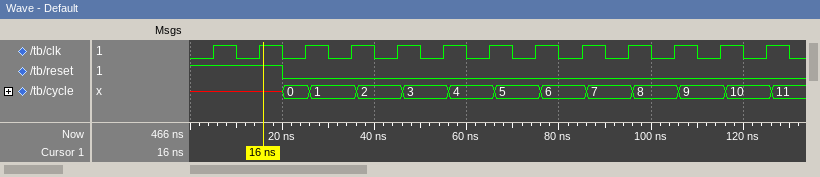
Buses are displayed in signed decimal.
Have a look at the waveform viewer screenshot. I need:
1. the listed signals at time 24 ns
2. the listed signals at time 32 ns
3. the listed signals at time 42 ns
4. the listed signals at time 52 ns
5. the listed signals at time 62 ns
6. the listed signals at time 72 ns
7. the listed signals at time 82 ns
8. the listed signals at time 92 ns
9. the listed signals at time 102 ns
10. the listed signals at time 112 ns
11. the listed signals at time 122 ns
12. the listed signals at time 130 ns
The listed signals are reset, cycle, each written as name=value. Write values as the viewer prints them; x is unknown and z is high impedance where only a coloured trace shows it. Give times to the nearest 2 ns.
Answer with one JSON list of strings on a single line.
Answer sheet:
["reset=0, cycle=0", "reset=0, cycle=1", "reset=0, cycle=2", "reset=0, cycle=3", "reset=0, cycle=4", "reset=0, cycle=5", "reset=0, cycle=6", "reset=0, cycle=7", "reset=0, cycle=8", "reset=0, cycle=9", "reset=0, cycle=10", "reset=0, cycle=11"]
